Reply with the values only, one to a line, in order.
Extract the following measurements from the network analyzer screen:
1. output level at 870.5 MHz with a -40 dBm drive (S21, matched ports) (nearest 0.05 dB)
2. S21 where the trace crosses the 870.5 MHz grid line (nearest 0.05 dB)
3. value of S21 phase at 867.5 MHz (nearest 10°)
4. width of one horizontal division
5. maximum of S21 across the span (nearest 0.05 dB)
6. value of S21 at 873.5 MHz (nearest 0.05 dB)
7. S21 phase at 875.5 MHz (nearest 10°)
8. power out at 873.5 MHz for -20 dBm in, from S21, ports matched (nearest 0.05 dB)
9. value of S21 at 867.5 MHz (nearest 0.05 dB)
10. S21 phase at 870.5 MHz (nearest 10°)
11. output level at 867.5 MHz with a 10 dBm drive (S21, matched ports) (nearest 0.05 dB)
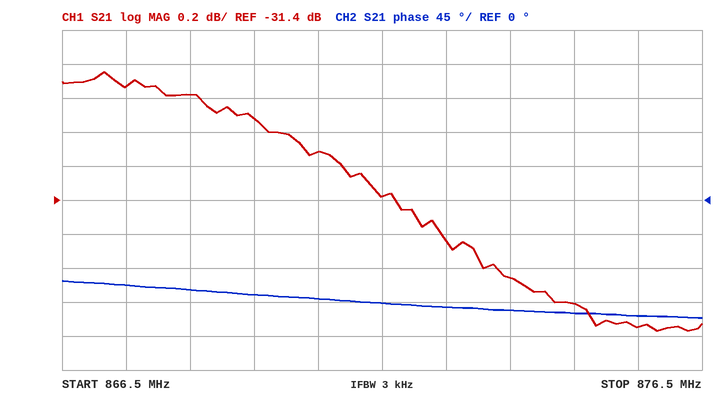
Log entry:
-71.10 dBm
-31.10 dB
-110°
1 MHz
-30.65 dB
-31.85 dB
-150°
-51.85 dBm
-30.75 dB
-130°
-20.75 dBm
